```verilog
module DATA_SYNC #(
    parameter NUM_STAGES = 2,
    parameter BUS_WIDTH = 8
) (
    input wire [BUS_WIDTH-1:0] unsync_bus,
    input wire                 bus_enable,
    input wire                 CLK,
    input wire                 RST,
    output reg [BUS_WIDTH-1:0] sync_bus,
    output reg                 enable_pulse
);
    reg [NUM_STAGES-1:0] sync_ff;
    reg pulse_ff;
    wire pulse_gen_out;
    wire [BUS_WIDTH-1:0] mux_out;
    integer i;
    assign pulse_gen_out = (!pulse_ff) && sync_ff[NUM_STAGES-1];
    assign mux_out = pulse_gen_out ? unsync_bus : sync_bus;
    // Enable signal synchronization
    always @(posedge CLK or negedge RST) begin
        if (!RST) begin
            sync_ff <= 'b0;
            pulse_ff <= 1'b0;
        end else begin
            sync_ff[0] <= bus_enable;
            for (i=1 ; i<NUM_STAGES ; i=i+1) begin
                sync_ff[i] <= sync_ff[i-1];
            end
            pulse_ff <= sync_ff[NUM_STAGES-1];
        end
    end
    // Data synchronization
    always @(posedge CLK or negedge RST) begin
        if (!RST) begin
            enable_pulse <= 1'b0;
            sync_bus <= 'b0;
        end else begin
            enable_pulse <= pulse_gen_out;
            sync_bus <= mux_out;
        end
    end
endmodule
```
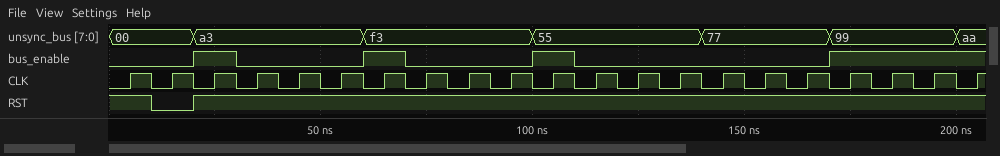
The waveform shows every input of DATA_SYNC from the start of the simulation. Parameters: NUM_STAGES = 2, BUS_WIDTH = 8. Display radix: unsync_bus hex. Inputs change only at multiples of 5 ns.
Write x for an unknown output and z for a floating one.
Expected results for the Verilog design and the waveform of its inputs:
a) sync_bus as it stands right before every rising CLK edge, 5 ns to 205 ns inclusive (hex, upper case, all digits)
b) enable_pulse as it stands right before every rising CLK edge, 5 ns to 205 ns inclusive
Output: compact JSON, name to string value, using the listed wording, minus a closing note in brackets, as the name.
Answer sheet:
{"sync_bus as it stands right before every rising CLK edge, 5 ns to 205 ns inclusive": "x, 00, 00, 00, 00, A3, A3, A3, A3, F3, F3, F3, F3, 55, 55, 55, 55, 55, 55, 55, 99", "enable_pulse as it stands right before every rising CLK edge, 5 ns to 205 ns inclusive": "x 0 0 0 0 1 0 0 0 1 0 0 0 1 0 0 0 0 0 0 1"}
